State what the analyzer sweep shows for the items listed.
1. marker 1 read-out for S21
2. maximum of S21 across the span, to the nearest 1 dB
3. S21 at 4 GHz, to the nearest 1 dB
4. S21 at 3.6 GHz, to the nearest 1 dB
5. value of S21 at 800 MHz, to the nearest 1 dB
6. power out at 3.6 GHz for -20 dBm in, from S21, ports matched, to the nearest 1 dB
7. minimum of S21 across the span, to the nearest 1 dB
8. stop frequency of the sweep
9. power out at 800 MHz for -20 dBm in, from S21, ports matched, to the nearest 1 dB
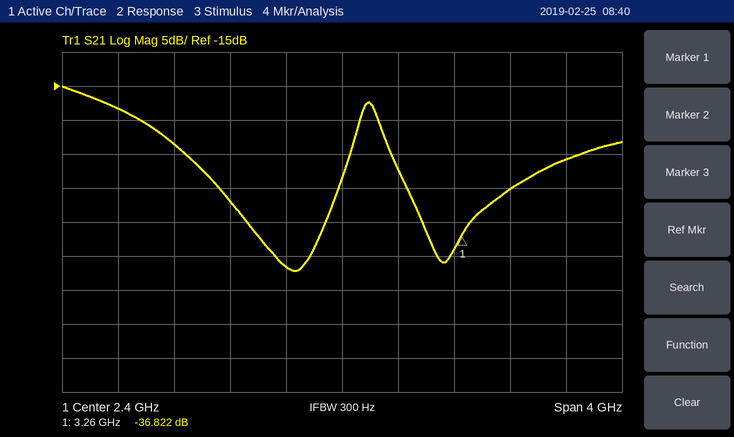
-36.822 dB
-15 dB
-26 dB
-30 dB
-18 dB
-50 dBm
-42 dB
4.4 GHz
-38 dBm
